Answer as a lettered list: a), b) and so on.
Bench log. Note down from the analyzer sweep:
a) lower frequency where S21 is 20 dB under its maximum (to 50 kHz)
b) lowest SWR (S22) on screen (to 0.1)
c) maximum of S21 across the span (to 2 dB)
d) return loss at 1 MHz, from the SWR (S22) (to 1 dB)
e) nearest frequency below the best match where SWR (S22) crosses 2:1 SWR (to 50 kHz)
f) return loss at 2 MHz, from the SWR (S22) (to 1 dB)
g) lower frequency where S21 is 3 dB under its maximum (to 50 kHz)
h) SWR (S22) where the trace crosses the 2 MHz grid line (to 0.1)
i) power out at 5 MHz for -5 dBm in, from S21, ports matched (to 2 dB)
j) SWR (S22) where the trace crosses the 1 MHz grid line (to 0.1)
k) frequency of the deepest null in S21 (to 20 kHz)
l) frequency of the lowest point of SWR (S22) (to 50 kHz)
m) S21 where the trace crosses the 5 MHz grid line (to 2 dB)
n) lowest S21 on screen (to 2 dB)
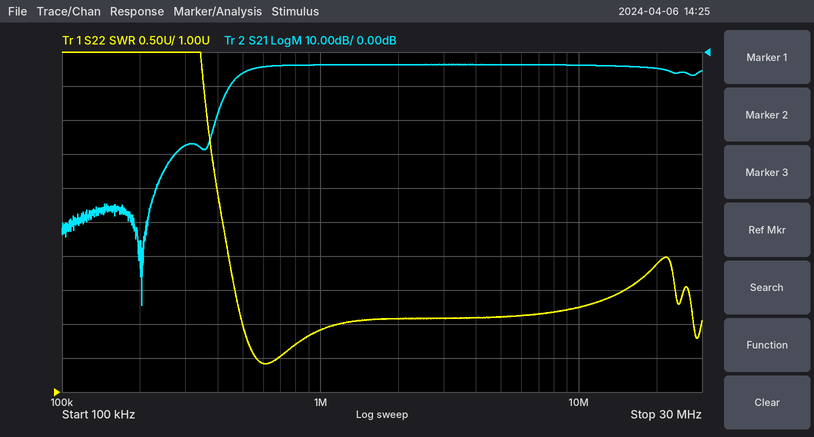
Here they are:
a) 400 kHz
b) 1.4
c) -4 dB
d) 10 dB
e) 500 kHz
f) 9 dB
g) 500 kHz
h) 2.1
i) -8 dBm
j) 1.9
k) 200 kHz
l) 600 kHz
m) -4 dB
n) -74 dB
